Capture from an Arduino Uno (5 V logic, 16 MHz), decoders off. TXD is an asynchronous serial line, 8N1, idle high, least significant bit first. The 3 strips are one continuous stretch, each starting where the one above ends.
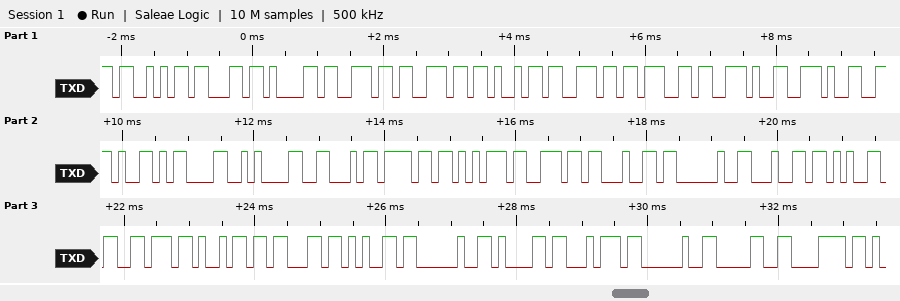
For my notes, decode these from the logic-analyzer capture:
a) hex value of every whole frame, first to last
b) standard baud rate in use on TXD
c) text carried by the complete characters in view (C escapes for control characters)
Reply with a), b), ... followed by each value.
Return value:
a) 0x53 0x63 0x61 0x6E 0x6E 0x69 0x6E 0x67 0x2E 0x2E 0x2E 0x0D 0x0A 0x46 0x6F 0x75 0x6E 0x64 0x20 0x64 0x65 0x76 0x69 0x63 0x65 0x20 0x61 0x74 0x20 0x30 0x78
b) 9600 baud
c) "Scanning...\r\nFound device at 0x"
